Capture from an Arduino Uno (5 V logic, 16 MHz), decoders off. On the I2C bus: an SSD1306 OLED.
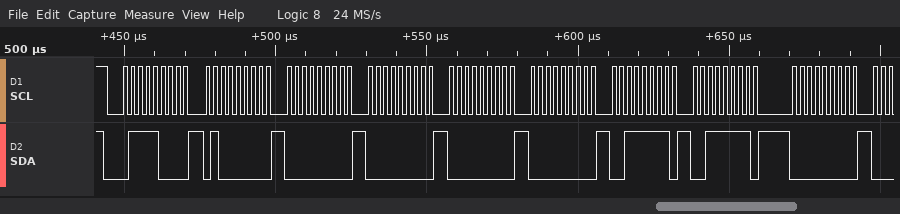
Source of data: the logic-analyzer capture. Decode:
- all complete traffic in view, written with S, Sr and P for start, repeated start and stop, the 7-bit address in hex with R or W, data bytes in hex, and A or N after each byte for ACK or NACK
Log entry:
S 3CW A 40 A 00 A 00 A 00 A 00 A 3F A 3F A 00 A
